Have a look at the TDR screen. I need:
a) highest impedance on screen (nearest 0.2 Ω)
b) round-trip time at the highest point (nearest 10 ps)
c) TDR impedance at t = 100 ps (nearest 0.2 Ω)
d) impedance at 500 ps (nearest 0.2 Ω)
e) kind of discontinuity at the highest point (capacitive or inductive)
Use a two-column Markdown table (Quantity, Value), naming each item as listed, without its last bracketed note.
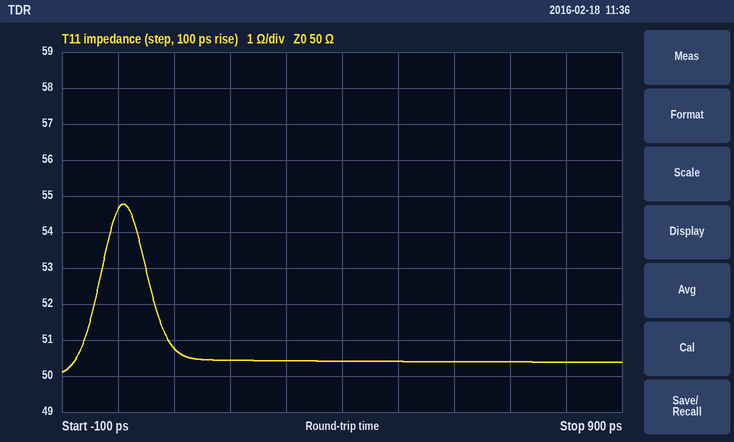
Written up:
| Quantity | Value |
|---|---|
| highest impedance on screen | 54.8 Ω |
| round-trip time at the highest point | 10 ps |
| TDR impedance at t = 100 ps | 50.8 Ω |
| impedance at 500 ps | 50.4 Ω |
| kind of discontinuity at the highest point | inductive |
